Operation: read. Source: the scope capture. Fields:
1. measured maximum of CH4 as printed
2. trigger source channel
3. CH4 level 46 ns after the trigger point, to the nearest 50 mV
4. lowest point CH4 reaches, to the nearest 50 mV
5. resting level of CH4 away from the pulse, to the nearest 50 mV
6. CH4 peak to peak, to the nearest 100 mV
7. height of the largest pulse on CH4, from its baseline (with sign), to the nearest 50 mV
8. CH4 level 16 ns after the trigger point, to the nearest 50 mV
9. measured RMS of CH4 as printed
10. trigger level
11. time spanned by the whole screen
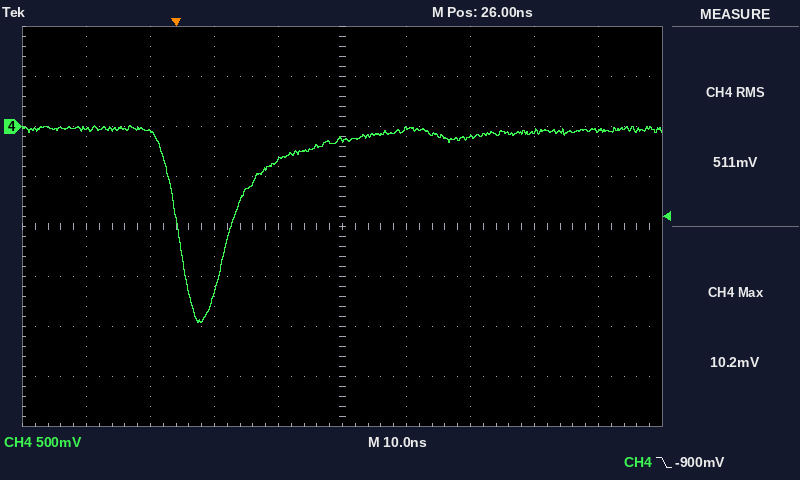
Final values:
10.2 mV
CH4
-100 mV
-1.95 V
-50 mV
2.00 V
-1.90 V
-350 mV
511 mV
-900 mV
100 ns
